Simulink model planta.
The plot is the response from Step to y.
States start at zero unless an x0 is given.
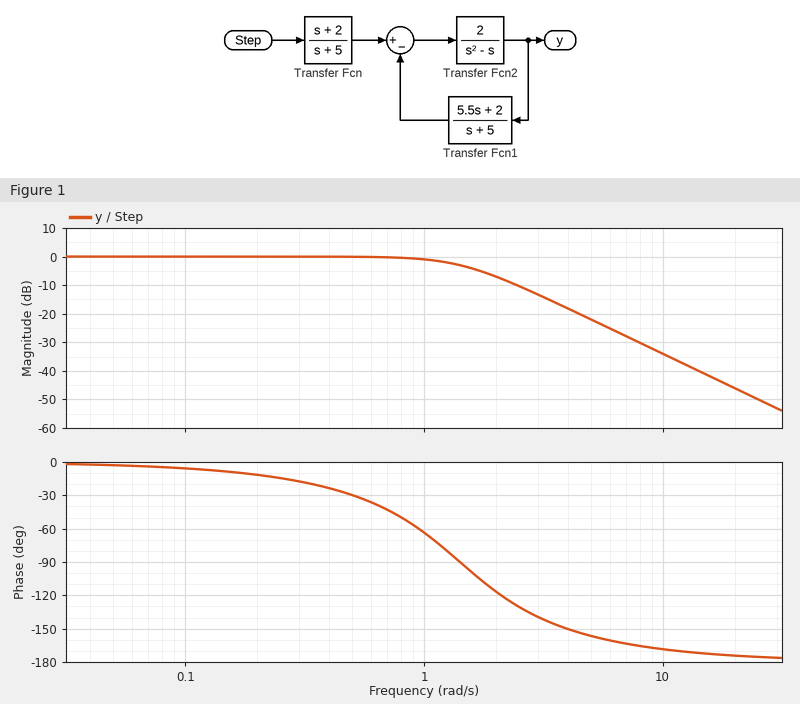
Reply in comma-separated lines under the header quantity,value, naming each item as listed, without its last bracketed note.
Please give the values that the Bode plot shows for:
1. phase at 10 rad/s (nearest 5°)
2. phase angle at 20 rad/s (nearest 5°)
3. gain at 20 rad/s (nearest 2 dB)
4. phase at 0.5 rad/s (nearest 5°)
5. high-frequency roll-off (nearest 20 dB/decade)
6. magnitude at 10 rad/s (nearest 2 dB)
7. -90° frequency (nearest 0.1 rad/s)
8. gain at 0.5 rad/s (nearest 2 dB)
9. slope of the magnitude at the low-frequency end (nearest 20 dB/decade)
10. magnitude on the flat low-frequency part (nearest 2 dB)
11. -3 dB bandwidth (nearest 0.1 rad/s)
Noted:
quantity,value
phase at 10 rad/s,-170°
phase angle at 20 rad/s,-175°
gain at 20 rad/s,-46 dB
phase at 0.5 rad/s,-30°
high-frequency roll-off,-40 dB/decade
magnitude at 10 rad/s,-34 dB
-90° frequency,1.4 rad/s
gain at 0.5 rad/s,0 dB
slope of the magnitude at the low-frequency end,0 dB/decade
magnitude on the flat low-frequency part,0 dB
-3 dB bandwidth,1.4 rad/s
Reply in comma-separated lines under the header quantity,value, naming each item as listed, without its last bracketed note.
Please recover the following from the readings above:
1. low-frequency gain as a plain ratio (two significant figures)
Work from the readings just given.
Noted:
quantity,value
low-frequency gain as a plain ratio,1.0
